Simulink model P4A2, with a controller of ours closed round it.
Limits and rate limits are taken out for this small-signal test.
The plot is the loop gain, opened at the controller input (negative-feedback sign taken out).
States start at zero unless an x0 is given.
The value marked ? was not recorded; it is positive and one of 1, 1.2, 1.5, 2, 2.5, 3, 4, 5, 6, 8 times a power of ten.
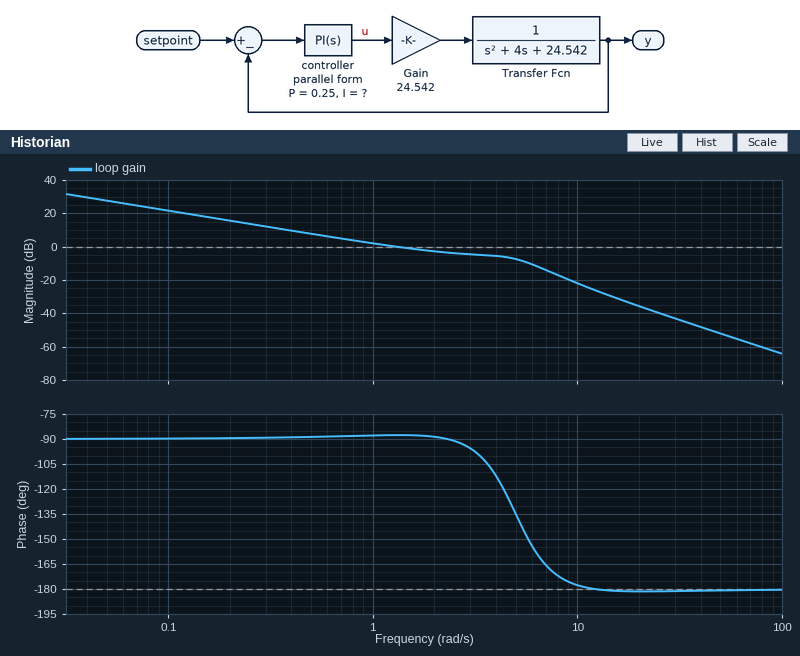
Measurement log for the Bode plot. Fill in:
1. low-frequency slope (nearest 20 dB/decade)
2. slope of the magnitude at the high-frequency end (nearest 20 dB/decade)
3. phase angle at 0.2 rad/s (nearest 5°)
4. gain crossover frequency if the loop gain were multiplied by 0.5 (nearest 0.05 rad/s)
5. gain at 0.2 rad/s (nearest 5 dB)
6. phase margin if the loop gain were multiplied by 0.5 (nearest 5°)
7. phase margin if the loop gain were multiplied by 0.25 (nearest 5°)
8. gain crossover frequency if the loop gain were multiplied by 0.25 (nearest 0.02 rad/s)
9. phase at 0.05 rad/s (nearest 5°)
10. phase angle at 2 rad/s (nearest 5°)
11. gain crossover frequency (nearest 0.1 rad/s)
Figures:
-20 dB/decade
-40 dB/decade
-90°
0.60 rad/s
15 dB
90°
90°
0.30 rad/s
-90°
-90°
1.3 rad/s
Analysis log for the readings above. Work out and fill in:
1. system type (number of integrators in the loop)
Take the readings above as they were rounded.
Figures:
1
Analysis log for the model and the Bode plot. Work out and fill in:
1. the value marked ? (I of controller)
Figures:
1.2
